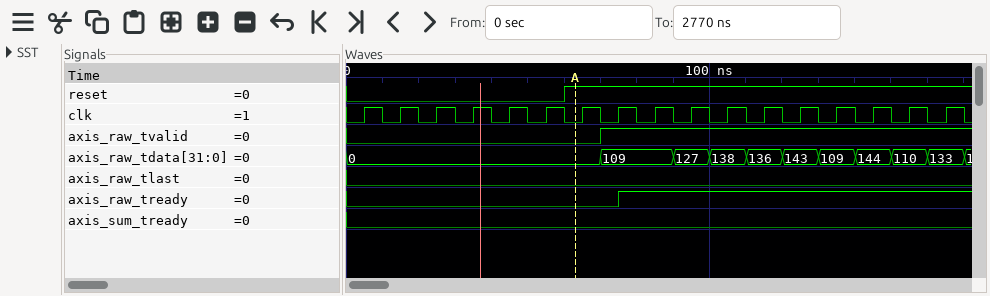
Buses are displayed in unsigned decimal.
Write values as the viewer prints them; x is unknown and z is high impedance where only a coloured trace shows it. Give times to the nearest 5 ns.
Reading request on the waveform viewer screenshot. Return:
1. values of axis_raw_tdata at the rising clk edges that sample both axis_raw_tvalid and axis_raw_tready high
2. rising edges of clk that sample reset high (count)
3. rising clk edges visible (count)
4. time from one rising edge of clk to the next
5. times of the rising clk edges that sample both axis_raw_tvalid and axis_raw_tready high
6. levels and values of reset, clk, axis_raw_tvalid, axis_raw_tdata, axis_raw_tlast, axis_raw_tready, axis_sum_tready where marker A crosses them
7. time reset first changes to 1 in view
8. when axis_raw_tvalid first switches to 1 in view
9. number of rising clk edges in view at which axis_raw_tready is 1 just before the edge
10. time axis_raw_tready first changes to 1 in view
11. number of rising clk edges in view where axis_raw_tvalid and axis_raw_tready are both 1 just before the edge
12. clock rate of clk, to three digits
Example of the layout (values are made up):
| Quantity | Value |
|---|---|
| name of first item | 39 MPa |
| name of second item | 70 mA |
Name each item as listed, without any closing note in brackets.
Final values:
| Quantity | Value |
|---|---|
| values of axis_raw_tdata at the rising clk edges that sample both axis_raw_tvalid and axis_raw_tready high | 109, 127, 138, 136, 143, 109, 144, 110, 133 |
| rising edges of clk that sample reset high | 11 |
| rising clk edges visible | 17 |
| time from one rising edge of clk to the next | 10 ns |
| times of the rising clk edges that sample both axis_raw_tvalid and axis_raw_tready high | 85 ns, 95 ns, 105 ns, 115 ns, 125 ns, 135 ns, 145 ns, 155 ns, 165 ns |
| levels and values of reset, clk, axis_raw_tvalid, axis_raw_tdata, axis_raw_tlast, axis_raw_tready, axis_sum_tready where marker A crosses them | reset=1, clk=0, axis_raw_tvalid=0, axis_raw_tdata=0, axis_raw_tlast=0, axis_raw_tready=0, axis_sum_tready=0 |
| time reset first changes to 1 in view | 60 ns |
| when axis_raw_tvalid first switches to 1 in view | 70 ns |
| number of rising clk edges in view at which axis_raw_tready is 1 just before the edge | 9 |
| time axis_raw_tready first changes to 1 in view | 75 ns |
| number of rising clk edges in view where axis_raw_tvalid and axis_raw_tready are both 1 just before the edge | 9 |
| clock rate of clk, to three digits | 100 MHz |
